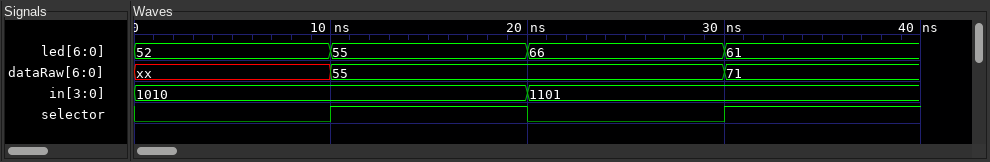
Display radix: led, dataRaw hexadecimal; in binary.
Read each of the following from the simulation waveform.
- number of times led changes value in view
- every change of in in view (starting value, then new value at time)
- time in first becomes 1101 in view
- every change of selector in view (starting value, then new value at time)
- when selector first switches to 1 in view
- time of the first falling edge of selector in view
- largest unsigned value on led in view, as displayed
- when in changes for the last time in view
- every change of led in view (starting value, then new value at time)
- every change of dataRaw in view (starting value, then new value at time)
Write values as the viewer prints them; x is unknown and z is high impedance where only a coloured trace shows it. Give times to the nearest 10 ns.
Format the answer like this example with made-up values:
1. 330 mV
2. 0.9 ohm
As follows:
1. 3
2. 1010, 1101 at 20 ns
3. 20 ns
4. 0, 1 at 10 ns, 0 at 20 ns, 1 at 30 ns
5. 10 ns
6. 20 ns
7. 66
8. 20 ns
9. 52, 55 at 10 ns, 66 at 20 ns, 61 at 30 ns
10. xx, 55 at 10 ns, 71 at 30 ns
